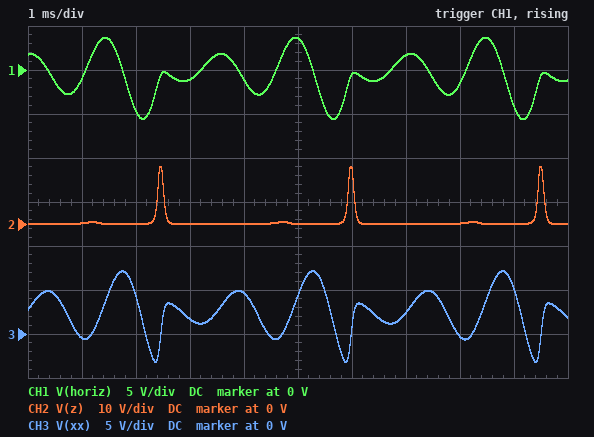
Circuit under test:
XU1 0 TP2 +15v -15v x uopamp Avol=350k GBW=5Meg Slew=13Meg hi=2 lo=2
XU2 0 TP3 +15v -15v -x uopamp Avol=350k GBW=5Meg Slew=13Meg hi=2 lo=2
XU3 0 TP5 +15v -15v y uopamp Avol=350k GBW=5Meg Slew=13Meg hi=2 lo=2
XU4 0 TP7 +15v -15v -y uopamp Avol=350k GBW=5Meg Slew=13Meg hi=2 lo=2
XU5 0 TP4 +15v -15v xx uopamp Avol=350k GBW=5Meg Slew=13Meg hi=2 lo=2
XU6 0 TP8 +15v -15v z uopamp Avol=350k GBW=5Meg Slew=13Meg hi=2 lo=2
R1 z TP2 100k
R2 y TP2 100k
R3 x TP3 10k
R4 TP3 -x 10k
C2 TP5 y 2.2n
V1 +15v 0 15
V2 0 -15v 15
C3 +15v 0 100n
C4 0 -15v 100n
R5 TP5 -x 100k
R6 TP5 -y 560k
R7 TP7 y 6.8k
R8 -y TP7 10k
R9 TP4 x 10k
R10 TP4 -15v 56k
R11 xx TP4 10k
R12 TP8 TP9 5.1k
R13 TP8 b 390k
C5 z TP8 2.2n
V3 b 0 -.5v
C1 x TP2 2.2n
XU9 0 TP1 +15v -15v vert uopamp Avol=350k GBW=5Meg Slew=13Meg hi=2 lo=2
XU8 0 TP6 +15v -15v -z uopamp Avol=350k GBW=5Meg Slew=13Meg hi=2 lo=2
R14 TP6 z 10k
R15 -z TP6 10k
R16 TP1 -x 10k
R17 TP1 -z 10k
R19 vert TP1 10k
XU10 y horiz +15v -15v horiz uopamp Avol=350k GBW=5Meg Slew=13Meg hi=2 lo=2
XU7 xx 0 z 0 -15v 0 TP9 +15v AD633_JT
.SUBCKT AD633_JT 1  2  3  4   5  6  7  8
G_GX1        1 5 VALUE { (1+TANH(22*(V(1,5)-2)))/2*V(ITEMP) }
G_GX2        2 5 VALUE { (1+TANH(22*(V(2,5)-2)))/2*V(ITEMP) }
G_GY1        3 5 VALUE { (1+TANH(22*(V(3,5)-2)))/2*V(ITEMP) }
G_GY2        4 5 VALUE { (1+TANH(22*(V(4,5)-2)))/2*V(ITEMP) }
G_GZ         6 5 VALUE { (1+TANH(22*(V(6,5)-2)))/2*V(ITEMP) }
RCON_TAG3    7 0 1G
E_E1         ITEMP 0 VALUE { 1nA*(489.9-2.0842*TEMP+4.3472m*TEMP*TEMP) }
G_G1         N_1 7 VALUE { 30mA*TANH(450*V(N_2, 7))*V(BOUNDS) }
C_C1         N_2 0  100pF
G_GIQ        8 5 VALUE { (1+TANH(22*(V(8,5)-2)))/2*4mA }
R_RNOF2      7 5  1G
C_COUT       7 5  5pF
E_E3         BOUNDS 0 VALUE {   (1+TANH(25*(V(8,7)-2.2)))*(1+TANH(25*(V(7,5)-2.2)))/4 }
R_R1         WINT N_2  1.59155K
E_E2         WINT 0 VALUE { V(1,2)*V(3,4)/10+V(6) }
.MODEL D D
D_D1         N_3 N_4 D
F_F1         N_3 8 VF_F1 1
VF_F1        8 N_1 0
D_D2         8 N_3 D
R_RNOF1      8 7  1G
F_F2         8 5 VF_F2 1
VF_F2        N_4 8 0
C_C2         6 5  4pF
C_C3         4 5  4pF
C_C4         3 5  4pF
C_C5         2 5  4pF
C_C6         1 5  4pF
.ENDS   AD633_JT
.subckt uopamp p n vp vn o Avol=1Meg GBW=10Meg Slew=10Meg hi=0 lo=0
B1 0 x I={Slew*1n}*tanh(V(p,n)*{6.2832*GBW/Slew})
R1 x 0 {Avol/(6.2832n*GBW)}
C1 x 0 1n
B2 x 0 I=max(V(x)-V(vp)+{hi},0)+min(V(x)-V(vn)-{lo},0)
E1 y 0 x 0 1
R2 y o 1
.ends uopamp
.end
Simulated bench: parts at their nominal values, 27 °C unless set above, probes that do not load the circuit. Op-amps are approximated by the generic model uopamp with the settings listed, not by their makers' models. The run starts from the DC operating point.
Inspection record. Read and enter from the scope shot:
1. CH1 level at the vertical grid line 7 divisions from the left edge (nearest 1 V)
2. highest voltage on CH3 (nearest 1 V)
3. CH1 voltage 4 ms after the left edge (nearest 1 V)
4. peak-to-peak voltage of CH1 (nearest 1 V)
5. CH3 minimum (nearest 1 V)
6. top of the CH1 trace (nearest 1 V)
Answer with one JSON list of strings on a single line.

["2 V", "7 V", "-1 V", "9 V", "-3 V", "4 V"]
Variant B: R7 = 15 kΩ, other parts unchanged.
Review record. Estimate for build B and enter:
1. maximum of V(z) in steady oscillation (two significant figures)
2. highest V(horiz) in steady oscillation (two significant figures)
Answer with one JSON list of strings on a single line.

["1.8 V", "3.2 V"]
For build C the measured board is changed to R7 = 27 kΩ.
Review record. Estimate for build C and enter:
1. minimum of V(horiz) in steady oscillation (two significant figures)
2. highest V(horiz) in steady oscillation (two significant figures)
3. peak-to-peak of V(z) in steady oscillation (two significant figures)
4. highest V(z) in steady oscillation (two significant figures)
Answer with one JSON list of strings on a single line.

["-3.6 V", "3.2 V", "830 mV", "840 mV"]
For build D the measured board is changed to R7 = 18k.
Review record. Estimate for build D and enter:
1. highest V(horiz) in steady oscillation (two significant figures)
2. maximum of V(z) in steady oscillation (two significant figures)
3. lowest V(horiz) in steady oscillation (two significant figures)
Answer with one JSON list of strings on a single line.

["3.2 V", "1.4 V", "-3.8 V"]
